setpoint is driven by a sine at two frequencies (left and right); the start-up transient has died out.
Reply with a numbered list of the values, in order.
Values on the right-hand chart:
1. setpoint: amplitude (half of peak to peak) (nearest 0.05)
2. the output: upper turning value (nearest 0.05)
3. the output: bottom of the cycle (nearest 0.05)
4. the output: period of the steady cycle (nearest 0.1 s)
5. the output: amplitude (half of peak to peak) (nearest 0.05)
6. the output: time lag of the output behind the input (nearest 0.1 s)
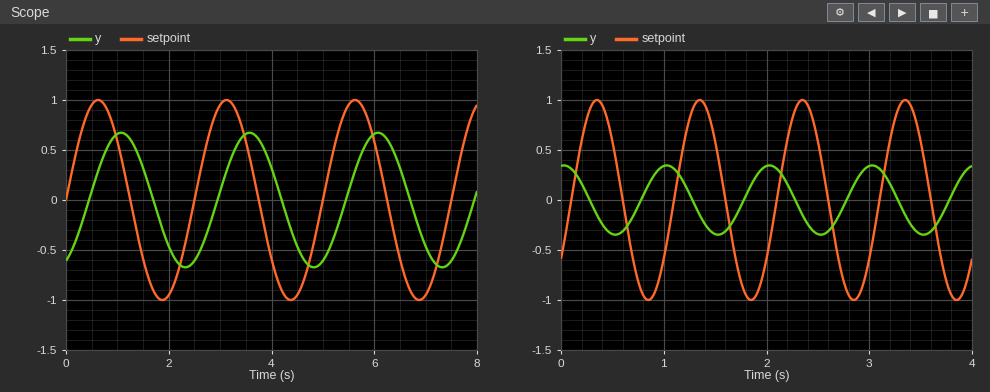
1. 1.00
2. 0.35
3. -0.35
4. 1.0 s
5. 0.35
6. 0.7 s
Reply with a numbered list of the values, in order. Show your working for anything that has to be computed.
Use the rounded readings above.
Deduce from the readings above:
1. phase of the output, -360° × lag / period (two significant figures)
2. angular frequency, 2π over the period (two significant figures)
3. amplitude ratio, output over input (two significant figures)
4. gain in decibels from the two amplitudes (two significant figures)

1. -360 × 0.7 / 1 = -250°
2. 2π / 1 = 6.3 rad/s
3. 0.35 / 1 = 0.35
4. 20 log10(0.35 / 1) = -9.1 dB
